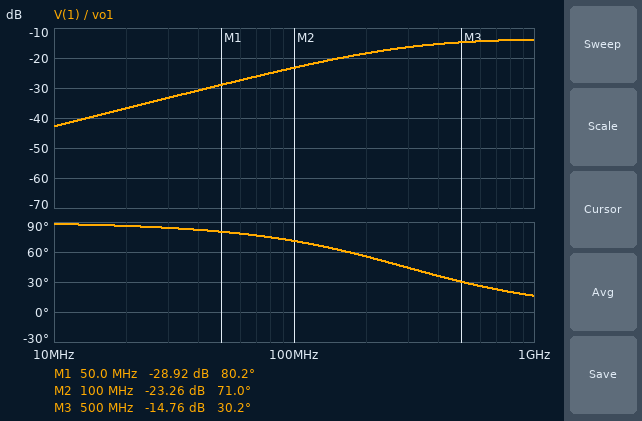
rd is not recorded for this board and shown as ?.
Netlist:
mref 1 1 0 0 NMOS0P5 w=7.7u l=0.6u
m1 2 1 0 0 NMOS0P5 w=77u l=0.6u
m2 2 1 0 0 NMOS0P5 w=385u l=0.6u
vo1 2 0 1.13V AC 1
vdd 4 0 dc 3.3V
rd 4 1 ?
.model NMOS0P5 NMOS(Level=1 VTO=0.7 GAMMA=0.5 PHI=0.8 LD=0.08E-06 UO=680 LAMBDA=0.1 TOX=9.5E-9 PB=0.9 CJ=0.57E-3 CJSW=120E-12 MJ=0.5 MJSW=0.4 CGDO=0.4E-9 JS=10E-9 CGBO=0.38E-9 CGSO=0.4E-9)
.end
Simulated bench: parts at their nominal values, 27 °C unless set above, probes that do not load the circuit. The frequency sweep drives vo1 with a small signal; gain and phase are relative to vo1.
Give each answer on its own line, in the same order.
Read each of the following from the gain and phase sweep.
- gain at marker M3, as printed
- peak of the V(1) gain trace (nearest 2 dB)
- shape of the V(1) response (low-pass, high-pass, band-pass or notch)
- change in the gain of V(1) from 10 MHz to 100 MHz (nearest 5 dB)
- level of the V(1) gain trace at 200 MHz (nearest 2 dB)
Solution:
-14.76 dB
-14 dB
high-pass
20 dB
-18 dB
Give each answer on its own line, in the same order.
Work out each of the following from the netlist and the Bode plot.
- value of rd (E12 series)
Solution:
10 kΩ
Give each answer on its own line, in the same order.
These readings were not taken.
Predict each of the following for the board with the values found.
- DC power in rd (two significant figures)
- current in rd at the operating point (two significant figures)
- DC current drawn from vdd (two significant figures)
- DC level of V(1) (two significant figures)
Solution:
520 µW
230 µA
230 µA
1.0 V
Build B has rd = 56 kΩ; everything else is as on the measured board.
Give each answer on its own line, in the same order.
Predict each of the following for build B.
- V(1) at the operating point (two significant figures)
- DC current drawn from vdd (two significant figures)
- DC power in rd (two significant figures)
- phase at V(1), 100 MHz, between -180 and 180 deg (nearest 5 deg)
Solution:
840 mV
44 µA
110 µW
50 deg
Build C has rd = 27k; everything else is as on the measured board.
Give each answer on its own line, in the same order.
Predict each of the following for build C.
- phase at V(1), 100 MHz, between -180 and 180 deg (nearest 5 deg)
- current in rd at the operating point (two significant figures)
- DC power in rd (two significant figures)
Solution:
60 deg
89 µA
210 µW
